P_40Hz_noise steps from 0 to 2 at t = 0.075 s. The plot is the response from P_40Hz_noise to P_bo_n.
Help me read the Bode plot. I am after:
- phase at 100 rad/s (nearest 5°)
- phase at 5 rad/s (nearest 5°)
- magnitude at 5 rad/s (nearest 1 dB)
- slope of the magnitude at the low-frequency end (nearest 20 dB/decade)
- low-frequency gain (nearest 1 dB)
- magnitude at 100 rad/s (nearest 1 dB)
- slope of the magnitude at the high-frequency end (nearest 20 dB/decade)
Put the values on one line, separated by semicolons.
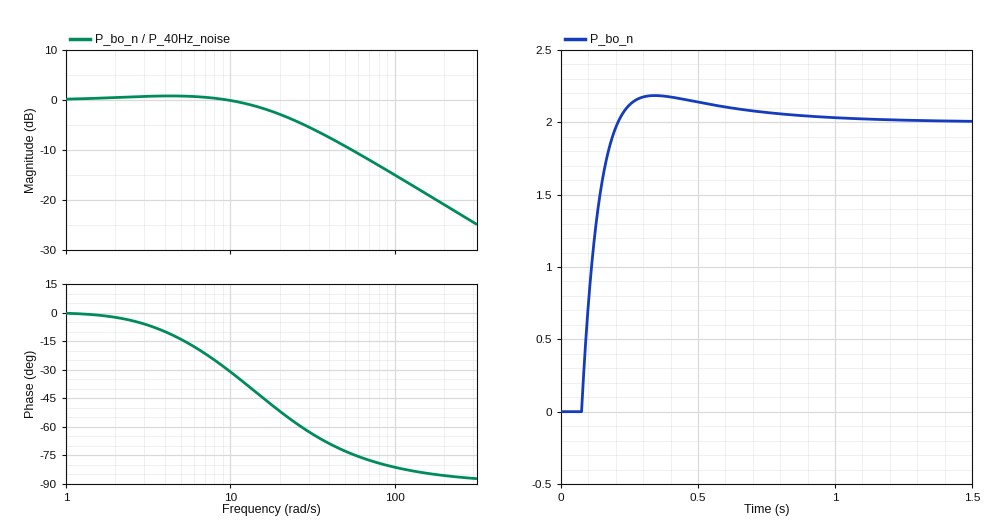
-80°; -15°; 1 dB; 0 dB/decade; 0 dB; -15 dB; -20 dB/decade
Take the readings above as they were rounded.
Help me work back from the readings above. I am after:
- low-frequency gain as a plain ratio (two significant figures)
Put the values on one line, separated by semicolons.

1.0
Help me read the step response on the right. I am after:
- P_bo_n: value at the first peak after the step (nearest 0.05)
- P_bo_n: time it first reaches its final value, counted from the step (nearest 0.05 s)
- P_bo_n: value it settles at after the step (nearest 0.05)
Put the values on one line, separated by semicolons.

2.20; 0.15 s; 2.00
